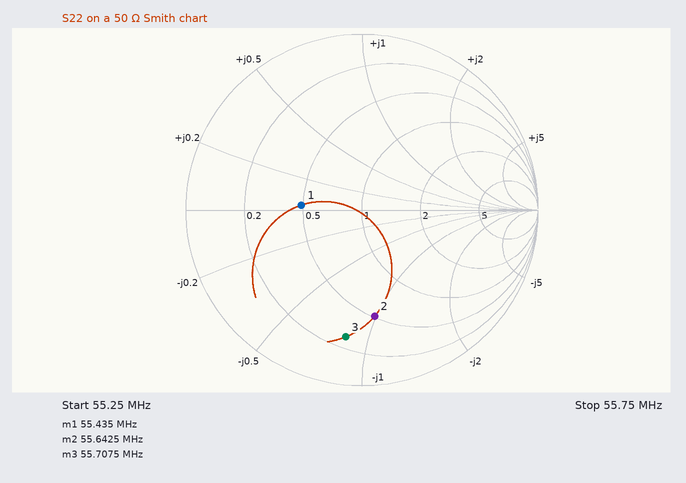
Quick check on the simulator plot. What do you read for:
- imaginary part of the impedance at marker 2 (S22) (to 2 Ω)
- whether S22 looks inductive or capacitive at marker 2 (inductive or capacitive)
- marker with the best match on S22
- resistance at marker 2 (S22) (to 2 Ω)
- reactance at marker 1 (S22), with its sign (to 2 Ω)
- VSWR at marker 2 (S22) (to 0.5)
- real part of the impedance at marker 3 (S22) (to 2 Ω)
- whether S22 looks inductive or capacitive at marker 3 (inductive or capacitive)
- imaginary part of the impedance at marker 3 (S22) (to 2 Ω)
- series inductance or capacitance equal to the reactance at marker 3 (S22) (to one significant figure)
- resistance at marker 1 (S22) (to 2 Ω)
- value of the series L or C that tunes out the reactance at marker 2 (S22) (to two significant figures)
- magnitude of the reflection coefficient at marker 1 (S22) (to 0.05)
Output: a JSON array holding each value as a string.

["-50 Ω", "capacitive", "marker 1", "26 Ω", "+2 Ω", "4.0", "14 Ω", "capacitive", "-42 Ω", "70 pF", "24 Ω", "140 nH", "0.35"]
